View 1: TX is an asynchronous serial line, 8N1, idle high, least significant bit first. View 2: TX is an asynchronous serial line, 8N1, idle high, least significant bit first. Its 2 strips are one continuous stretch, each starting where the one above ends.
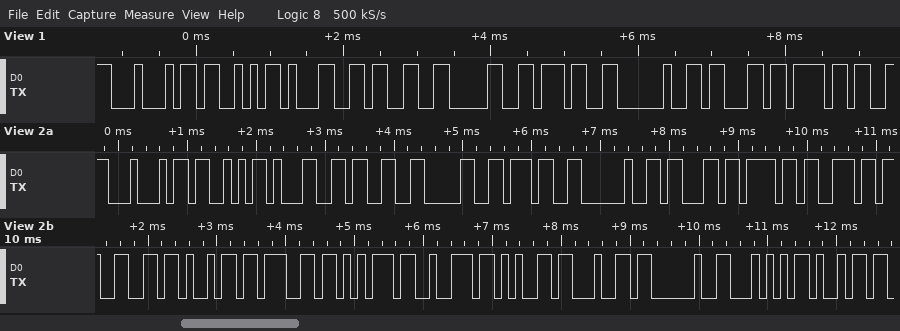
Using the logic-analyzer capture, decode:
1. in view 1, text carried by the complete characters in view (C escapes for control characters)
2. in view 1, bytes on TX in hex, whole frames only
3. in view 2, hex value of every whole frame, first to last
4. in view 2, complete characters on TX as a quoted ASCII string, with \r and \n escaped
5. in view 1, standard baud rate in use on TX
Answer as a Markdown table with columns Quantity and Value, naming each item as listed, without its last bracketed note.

| Quantity | Value |
|---|---|
| in view 1, text carried by the complete characters in view | "DS1307 co" |
| in view 1, bytes on TX in hex, whole frames only | 44 53 31 33 30 37 20 63 6F |
| in view 2, hex value of every whole frame, first to last | 0x44 0x53 0x31 0x33 0x30 0x37 0x20 0x63 0x6F 0x6E 0x66 0x69 0x67 0x75 0x72 0x65 0x64 0x20 0x54 0x69 |
| in view 2, complete characters on TX as a quoted ASCII string, with \r and \n escaped | "DS1307 configured Ti" |
| in view 1, standard baud rate in use on TX | 9600 baud |
